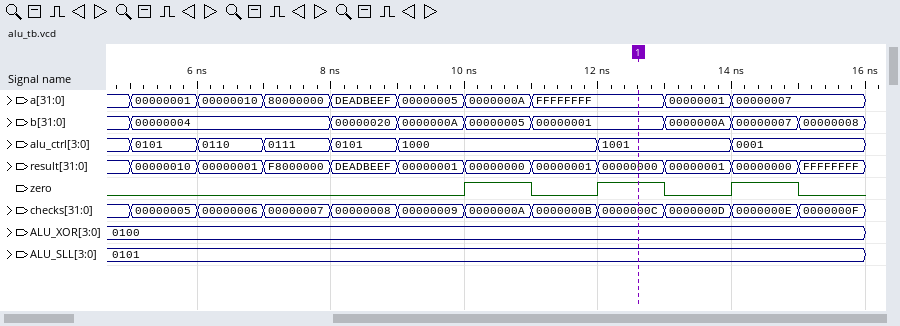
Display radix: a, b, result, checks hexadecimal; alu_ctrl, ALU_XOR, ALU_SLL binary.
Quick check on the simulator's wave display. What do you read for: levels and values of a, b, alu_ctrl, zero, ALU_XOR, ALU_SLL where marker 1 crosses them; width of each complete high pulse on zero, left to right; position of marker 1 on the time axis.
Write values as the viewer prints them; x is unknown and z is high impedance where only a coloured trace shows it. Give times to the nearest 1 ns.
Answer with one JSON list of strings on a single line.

["a=FFFFFFFF, b=00000001, alu_ctrl=1001, zero=1, ALU_XOR=0100, ALU_SLL=0101", "1 ns, 1 ns, 1 ns", "13 ns"]
